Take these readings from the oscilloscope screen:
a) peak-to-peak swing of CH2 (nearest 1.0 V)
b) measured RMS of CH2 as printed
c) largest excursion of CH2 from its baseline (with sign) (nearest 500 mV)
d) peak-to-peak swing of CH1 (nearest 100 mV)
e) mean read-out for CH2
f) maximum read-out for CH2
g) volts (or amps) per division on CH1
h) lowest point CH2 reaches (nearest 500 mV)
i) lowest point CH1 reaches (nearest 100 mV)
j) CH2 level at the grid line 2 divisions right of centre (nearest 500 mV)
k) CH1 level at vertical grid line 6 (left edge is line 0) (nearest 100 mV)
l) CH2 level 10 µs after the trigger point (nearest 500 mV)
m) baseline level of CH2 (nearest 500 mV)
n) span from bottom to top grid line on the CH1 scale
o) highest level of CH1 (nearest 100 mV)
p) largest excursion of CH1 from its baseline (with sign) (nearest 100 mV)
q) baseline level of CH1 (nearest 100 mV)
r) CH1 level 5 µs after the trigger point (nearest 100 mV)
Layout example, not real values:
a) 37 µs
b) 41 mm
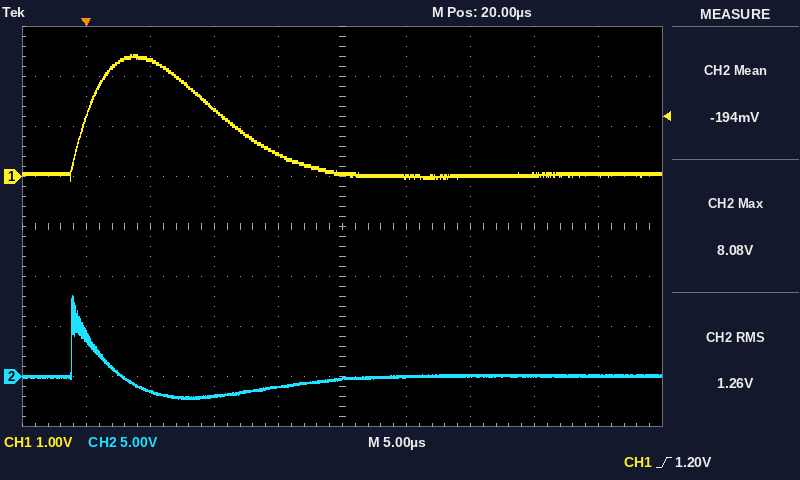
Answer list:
a) 10.0 V
b) 1.26 V
c) +8.0 V
d) 2.5 V
e) -194 mV
f) 8.08 V
g) 1 V
h) -2.0 V
i) -100 mV
j) 0.0 V
k) 0.0 V
l) -2.0 V
m) 0.0 V
n) 8 V
o) 2.4 V
p) +2.4 V
q) 0.0 V
r) 2.3 V
